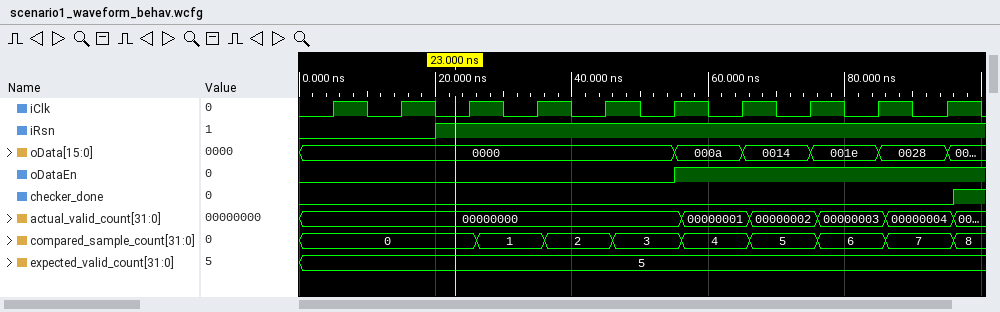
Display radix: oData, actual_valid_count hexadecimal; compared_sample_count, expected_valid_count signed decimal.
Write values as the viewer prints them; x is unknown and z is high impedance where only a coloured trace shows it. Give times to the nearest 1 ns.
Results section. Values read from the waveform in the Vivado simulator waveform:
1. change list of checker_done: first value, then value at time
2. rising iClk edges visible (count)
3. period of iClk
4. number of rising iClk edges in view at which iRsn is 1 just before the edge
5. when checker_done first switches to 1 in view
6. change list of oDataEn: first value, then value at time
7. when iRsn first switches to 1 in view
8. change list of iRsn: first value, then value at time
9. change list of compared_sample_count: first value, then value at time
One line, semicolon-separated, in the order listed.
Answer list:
0, 1 at 96 ns; 10; 10 ns; 8; 96 ns; 0, 1 at 55 ns; 20 ns; 0, 1 at 20 ns; 0, 1 at 26 ns, 2 at 36 ns, 3 at 46 ns, 4 at 56 ns, 5 at 66 ns, 6 at 76 ns, 7 at 86 ns, 8 at 96 ns
